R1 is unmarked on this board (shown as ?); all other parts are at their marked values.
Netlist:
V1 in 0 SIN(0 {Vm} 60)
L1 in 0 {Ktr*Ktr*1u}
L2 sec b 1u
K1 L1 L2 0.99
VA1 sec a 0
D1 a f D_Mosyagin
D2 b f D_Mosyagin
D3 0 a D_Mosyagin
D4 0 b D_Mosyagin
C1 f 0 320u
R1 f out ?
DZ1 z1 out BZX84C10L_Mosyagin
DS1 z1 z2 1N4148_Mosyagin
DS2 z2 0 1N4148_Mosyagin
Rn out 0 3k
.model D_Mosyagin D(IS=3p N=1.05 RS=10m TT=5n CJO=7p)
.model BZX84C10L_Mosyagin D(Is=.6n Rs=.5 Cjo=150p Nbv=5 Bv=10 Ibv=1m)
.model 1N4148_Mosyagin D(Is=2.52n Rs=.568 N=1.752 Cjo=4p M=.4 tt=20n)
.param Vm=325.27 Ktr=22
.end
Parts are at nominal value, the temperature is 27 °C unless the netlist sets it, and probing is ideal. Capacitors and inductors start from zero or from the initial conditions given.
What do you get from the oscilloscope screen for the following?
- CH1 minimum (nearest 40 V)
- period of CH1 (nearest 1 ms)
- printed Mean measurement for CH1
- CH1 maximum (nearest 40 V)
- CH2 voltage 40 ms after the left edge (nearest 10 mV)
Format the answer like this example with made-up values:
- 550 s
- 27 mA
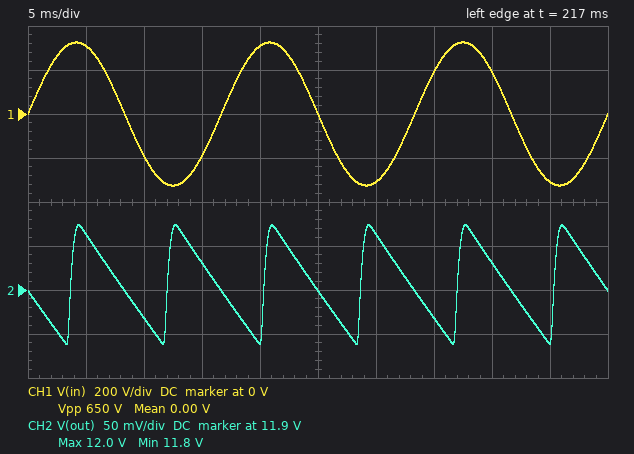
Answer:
- -320 V
- 17 ms
- 0.00 V
- 320 V
- 11.93 V
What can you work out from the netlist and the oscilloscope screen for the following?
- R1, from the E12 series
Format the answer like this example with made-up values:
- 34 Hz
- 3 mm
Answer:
- 39 Ω
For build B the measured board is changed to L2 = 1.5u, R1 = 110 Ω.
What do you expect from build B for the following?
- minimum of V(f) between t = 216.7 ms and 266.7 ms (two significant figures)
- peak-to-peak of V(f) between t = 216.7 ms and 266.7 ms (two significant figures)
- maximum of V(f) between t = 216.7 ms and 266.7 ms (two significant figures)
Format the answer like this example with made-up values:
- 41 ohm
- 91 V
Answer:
- 16 V
- 850 mV
- 17 V
